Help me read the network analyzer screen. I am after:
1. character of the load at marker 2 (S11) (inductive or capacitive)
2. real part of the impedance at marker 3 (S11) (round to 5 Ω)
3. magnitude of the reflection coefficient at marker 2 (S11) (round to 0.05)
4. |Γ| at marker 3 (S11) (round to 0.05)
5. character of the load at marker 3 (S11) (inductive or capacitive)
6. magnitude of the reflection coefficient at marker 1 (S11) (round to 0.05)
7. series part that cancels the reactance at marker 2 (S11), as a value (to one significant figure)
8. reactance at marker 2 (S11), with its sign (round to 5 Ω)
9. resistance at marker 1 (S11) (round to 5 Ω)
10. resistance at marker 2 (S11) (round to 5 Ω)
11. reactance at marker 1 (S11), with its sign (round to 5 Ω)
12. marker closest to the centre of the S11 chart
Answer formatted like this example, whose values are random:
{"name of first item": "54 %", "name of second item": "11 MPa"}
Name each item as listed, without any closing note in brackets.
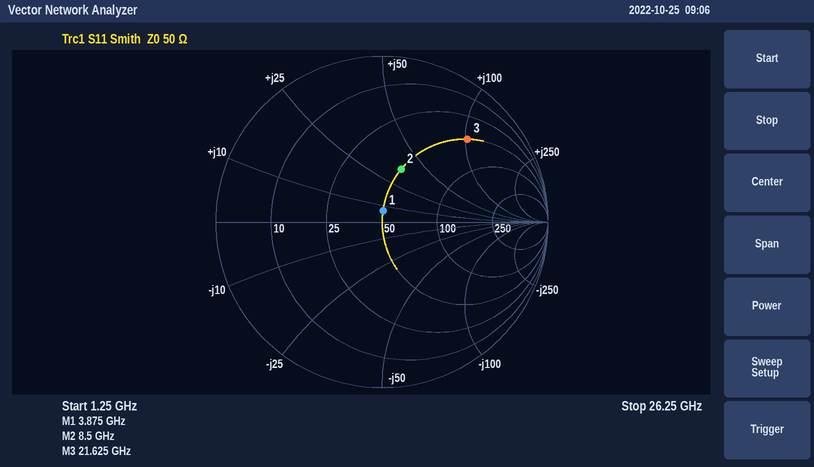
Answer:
{"character of the load at marker 2 (S11)": "inductive", "real part of the impedance at marker 3 (S11)": "50 Ω", "magnitude of the reflection coefficient at marker 2 (S11)": "0.35", "|Γ| at marker 3 (S11)": "0.70", "character of the load at marker 3 (S11)": "inductive", "magnitude of the reflection coefficient at marker 1 (S11)": "0.05", "series part that cancels the reactance at marker 2 (S11), as a value": "500 fF", "reactance at marker 2 (S11), with its sign": "+35 Ω", "resistance at marker 1 (S11)": "50 Ω", "resistance at marker 2 (S11)": "50 Ω", "reactance at marker 1 (S11), with its sign": "+5 Ω", "marker closest to the centre of the S11 chart": "marker 1"}
